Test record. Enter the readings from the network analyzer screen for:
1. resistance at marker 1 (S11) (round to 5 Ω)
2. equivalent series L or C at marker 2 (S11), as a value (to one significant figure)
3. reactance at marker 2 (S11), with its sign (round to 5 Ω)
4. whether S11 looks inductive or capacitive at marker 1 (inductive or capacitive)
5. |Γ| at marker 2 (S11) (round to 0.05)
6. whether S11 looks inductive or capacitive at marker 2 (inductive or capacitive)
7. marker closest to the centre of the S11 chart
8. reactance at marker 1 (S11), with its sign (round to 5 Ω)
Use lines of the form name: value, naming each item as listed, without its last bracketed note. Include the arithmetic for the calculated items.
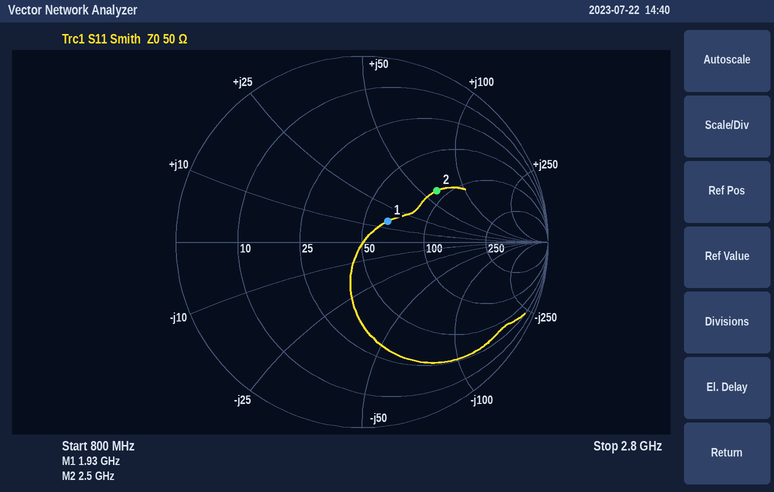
resistance at marker 1 (S11): 65 Ω
equivalent series L or C at marker 2 (S11), as a value: L = 65 Ω/(2π × 2.5 GHz) ≈ 4 nH
reactance at marker 2 (S11), with its sign: +65 Ω
whether S11 looks inductive or capacitive at marker 1: inductive
|Γ| at marker 2 (S11): 0.50
whether S11 looks inductive or capacitive at marker 2: inductive
marker closest to the centre of the S11 chart: marker 1
reactance at marker 1 (S11), with its sign: +15 Ω
